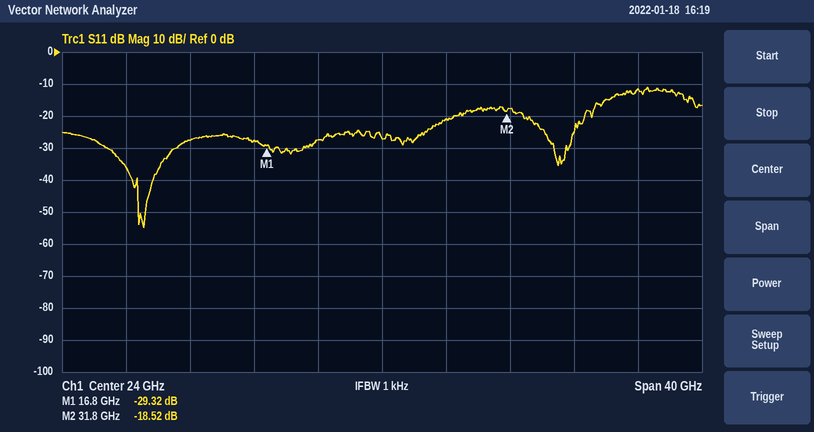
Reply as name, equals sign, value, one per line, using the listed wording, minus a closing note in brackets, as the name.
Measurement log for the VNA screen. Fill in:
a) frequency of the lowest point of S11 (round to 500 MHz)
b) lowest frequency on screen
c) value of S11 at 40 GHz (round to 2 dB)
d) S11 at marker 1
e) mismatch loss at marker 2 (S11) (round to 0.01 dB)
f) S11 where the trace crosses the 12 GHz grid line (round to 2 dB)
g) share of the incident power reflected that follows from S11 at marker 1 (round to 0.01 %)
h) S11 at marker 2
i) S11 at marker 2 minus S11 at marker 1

frequency of the lowest point of S11 = 9.0 GHz
lowest frequency on screen = 4 GHz
value of S11 at 40 GHz = -12 dB
S11 at marker 1 = -29.32 dB
mismatch loss at marker 2 (S11) = 0.06 dB
S11 where the trace crosses the 12 GHz grid line = -28 dB
share of the incident power reflected that follows from S11 at marker 1 = 0.12 %
S11 at marker 2 = -18.52 dB
S11 at marker 2 minus S11 at marker 1 = 10.80 dB
